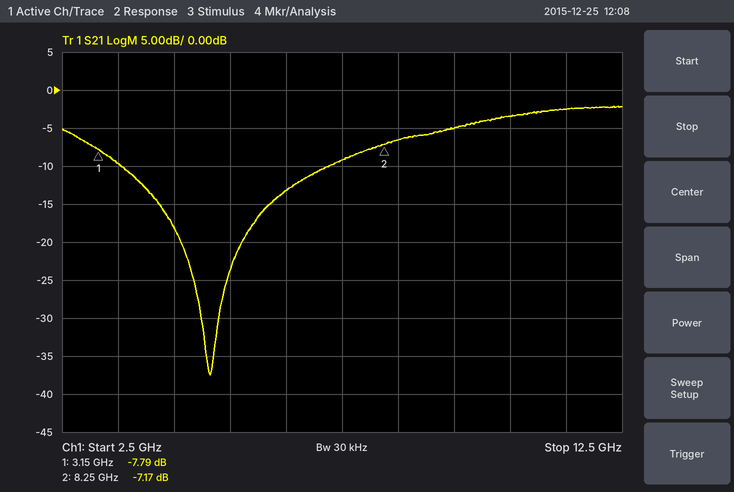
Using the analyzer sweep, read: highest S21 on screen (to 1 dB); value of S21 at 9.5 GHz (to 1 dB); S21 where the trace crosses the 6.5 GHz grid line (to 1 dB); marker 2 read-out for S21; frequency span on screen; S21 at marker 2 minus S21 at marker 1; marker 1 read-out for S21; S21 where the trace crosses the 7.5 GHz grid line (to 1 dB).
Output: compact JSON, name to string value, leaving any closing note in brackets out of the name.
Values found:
{"highest S21 on screen": "-2 dB", "value of S21 at 9.5 GHz": "-5 dB", "S21 where the trace crosses the 6.5 GHz grid line": "-13 dB", "marker 2 read-out for S21": "-7.17 dB", "frequency span on screen": "10 GHz", "S21 at marker 2 minus S21 at marker 1": "0.62 dB", "marker 1 read-out for S21": "-7.79 dB", "S21 where the trace crosses the 7.5 GHz grid line": "-9 dB"}
